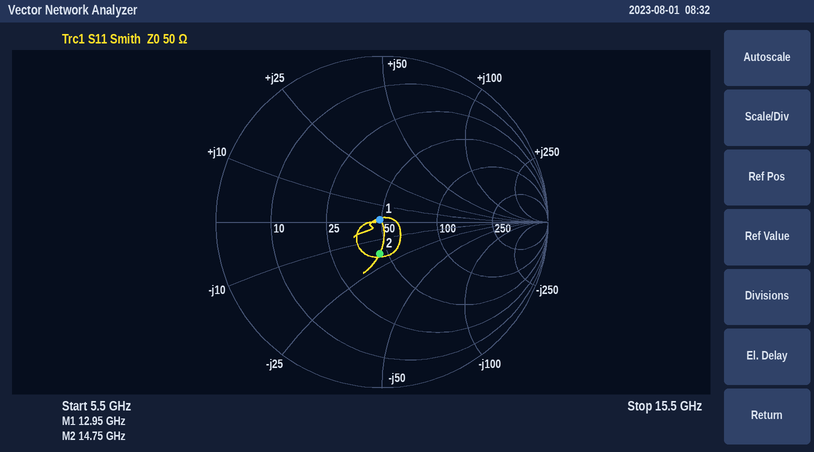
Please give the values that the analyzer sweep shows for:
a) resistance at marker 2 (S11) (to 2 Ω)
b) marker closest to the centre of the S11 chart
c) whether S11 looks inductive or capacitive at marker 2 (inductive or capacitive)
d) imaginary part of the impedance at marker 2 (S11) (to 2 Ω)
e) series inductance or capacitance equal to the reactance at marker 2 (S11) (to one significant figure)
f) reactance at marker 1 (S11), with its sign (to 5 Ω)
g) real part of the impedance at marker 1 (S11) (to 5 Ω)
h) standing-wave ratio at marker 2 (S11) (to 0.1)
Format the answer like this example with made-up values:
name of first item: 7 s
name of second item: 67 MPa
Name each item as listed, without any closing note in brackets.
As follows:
resistance at marker 2 (S11): 46 Ω
marker closest to the centre of the S11 chart: marker 1
whether S11 looks inductive or capacitive at marker 2: capacitive
imaginary part of the impedance at marker 2 (S11): -18 Ω
series inductance or capacitance equal to the reactance at marker 2 (S11): 600 fF
reactance at marker 1 (S11), with its sign: 0 Ω
real part of the impedance at marker 1 (S11): 50 Ω
standing-wave ratio at marker 2 (S11): 1.5
